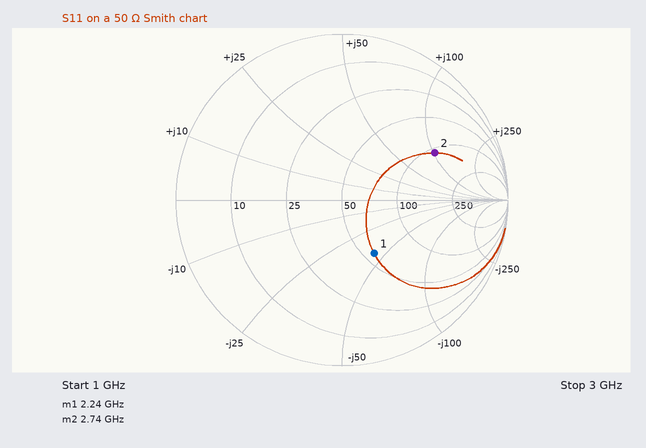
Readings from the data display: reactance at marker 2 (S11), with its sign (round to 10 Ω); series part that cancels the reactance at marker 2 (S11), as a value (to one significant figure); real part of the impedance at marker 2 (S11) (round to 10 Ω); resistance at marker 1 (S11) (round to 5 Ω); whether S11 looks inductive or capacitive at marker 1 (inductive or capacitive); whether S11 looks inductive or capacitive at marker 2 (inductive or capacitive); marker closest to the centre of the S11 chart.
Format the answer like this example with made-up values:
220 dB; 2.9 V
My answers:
+100 Ω; 600 fF; 110 Ω; 55 Ω; capacitive; inductive; marker 1
